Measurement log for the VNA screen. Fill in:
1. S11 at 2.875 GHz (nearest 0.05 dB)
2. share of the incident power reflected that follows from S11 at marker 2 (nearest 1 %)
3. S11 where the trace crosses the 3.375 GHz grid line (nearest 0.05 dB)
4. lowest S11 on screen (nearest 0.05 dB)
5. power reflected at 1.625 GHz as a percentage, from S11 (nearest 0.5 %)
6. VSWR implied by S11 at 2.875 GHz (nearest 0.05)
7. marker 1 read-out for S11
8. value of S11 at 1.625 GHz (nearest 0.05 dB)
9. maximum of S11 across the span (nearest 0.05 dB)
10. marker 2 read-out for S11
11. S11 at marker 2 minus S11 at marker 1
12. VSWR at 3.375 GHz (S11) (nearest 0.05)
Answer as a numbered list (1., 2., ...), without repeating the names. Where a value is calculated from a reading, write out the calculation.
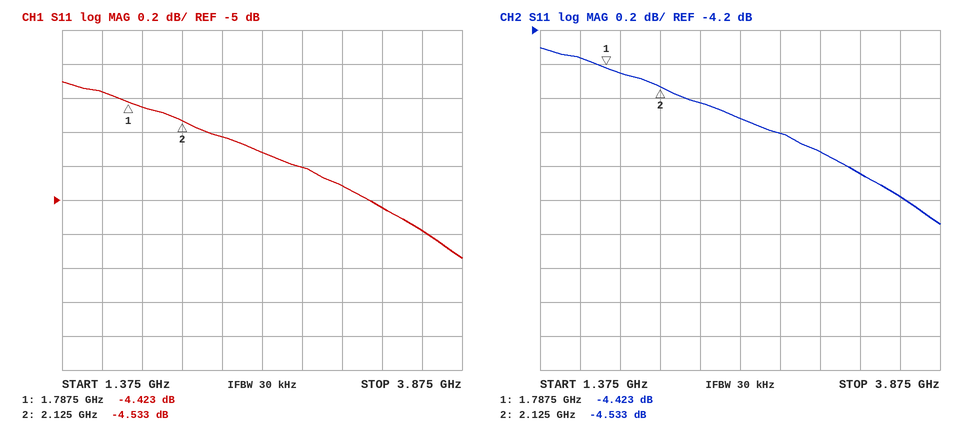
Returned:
1. -4.80 dB
2. 10^(-4.533/10) ≈ 35 %
3. -5.05 dB
4. -5.35 dB
5. 10^(-4.35/10) ≈ 36.7 %, so 36.5 % to the nearest 0.5 %
6. |Γ| = 10^(-4.8/20) = 0.5754; VSWR = (1 + 0.5754)/(1 − 0.5754) ≈ 3.71, so 3.70 to the nearest 0.05
7. -4.423 dB
8. -4.35 dB
9. -4.30 dB
10. -4.533 dB
11. -4.533 − (-4.423) = -0.110 dB
12. |Γ| = 10^(-5.05/20) = 0.5591; VSWR = (1 + 0.5591)/(1 − 0.5591) ≈ 3.54, so 3.55 to the nearest 0.05
